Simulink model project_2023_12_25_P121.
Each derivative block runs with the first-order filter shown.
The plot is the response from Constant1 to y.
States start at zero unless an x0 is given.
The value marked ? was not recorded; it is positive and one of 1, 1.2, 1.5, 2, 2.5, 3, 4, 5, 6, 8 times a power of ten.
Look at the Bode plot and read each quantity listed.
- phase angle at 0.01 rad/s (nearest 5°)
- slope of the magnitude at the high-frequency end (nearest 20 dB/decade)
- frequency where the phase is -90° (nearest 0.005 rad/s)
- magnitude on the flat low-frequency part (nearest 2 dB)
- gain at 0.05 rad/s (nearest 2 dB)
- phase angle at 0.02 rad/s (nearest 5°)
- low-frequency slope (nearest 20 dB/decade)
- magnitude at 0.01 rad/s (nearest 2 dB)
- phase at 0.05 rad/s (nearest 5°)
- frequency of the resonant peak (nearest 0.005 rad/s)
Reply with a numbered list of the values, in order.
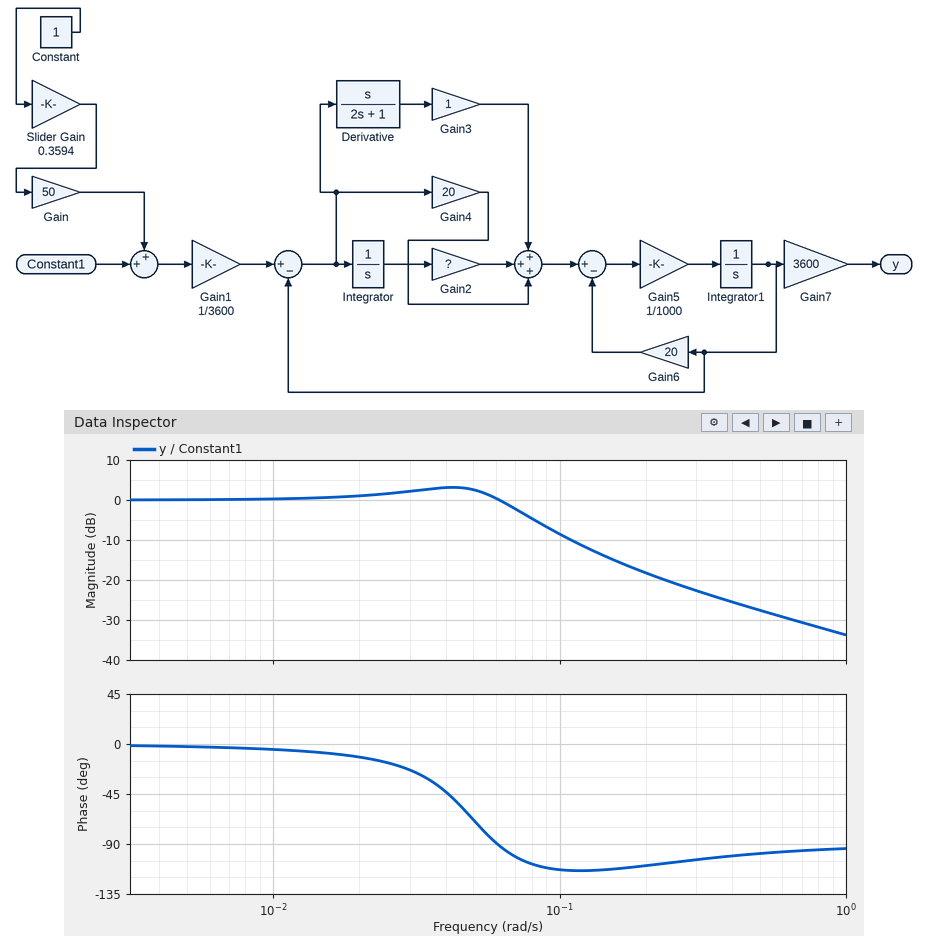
1. -5°
2. -20 dB/decade
3. 0.060 rad/s
4. 0 dB
5. 2 dB
6. -10°
7. 0 dB/decade
8. 0 dB
9. -70°
10. 0.040 rad/s
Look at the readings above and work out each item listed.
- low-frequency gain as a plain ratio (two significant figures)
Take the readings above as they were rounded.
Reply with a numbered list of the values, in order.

1. 1.0
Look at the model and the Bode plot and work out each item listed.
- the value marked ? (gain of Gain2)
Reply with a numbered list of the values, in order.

1. 2.5
